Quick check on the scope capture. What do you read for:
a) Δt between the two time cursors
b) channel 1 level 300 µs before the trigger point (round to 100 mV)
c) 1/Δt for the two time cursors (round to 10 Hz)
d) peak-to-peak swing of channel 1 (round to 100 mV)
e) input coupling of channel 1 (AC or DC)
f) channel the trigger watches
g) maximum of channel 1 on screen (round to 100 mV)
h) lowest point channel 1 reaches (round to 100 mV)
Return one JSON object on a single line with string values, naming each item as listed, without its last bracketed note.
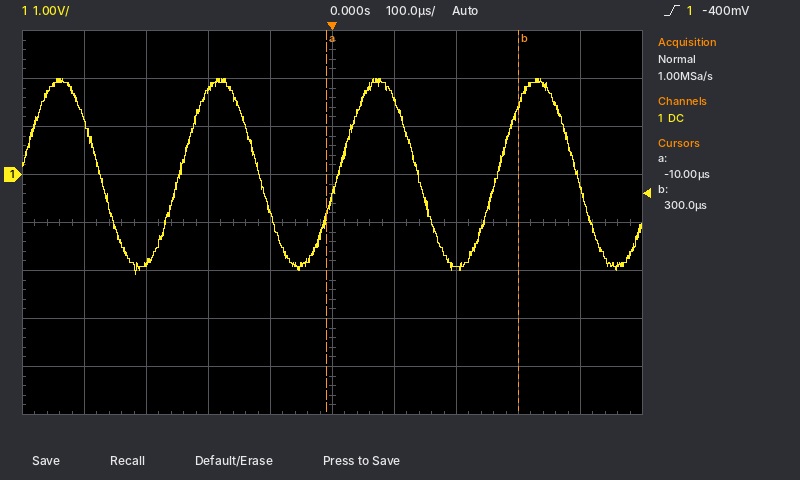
{"Δt between the two time cursors": "310 µs", "channel 1 level 300 µs before the trigger point": "-1.8 V", "1/Δt for the two time cursors": "3.23 kHz", "peak-to-peak swing of channel 1": "4.1 V", "input coupling of channel 1": "DC", "channel the trigger watches": "channel 1", "maximum of channel 1 on screen": "2.0 V", "lowest point channel 1 reaches": "-2.1 V"}
